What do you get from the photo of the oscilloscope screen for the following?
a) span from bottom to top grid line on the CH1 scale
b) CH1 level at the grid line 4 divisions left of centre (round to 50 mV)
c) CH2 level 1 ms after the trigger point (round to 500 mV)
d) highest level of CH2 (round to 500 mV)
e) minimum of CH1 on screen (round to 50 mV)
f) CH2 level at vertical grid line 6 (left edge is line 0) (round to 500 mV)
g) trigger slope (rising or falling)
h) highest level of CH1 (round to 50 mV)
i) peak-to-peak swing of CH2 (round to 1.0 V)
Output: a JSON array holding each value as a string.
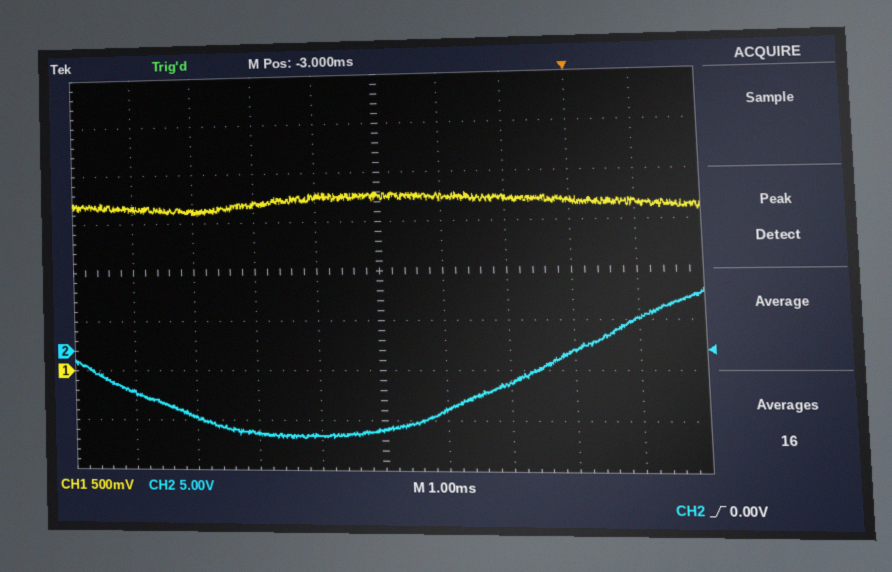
["4 V", "1.65 V", "3.5 V", "6.0 V", "1.60 V", "-6.0 V", "rising", "1.80 V", "15.0 V"]
